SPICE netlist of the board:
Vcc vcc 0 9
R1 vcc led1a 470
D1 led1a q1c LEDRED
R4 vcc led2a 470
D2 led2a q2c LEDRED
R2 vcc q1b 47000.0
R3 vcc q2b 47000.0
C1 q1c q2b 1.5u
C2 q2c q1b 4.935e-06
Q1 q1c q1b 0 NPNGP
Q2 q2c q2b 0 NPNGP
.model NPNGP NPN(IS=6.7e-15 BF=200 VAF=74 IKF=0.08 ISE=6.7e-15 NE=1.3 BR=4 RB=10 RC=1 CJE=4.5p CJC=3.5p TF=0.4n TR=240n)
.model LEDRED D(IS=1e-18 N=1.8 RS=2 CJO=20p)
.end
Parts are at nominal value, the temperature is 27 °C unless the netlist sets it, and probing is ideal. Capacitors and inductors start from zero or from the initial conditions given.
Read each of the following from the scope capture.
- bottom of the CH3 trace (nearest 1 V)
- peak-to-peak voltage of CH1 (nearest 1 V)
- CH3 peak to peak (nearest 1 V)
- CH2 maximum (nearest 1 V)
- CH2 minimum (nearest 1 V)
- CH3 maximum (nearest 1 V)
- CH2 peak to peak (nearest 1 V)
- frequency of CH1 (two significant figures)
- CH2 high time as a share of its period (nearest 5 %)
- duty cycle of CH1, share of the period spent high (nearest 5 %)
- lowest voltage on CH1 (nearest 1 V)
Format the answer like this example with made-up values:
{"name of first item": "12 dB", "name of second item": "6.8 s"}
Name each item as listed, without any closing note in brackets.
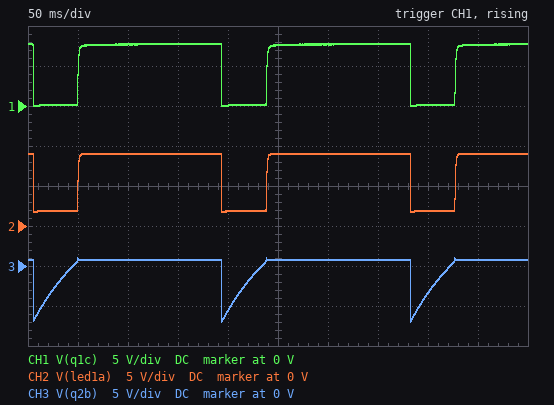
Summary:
{"bottom of the CH3 trace": "-7 V", "peak-to-peak voltage of CH1": "8 V", "CH3 peak to peak": "8 V", "CH2 maximum": "9 V", "CH2 minimum": "2 V", "CH3 maximum": "1 V", "CH2 peak to peak": "7 V", "frequency of CH1": "5.3 Hz", "CH2 high time as a share of its period": "75 %", "duty cycle of CH1, share of the period spent high": "75 %", "lowest voltage on CH1": "0 V"}
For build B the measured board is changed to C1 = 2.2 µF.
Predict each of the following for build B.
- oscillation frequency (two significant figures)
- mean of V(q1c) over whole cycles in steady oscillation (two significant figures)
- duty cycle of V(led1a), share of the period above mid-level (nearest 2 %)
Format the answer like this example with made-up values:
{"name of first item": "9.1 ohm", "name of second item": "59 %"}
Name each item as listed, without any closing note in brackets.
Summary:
{"oscillation frequency": "4.8 Hz", "mean of V(q1c) over whole cycles in steady oscillation": "5.3 V", "duty cycle of V(led1a), share of the period above mid-level": "68 %"}
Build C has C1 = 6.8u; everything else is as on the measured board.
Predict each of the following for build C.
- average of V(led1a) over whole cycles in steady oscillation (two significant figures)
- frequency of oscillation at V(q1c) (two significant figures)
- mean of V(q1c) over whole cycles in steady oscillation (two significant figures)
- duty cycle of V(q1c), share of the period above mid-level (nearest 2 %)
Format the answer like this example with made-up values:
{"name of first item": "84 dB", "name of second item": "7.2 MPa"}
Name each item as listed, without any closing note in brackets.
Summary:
{"average of V(led1a) over whole cycles in steady oscillation": "4.8 V", "frequency of oscillation at V(q1c)": "2.9 Hz", "mean of V(q1c) over whole cycles in steady oscillation": "3.2 V", "duty cycle of V(q1c), share of the period above mid-level": "42 %"}
